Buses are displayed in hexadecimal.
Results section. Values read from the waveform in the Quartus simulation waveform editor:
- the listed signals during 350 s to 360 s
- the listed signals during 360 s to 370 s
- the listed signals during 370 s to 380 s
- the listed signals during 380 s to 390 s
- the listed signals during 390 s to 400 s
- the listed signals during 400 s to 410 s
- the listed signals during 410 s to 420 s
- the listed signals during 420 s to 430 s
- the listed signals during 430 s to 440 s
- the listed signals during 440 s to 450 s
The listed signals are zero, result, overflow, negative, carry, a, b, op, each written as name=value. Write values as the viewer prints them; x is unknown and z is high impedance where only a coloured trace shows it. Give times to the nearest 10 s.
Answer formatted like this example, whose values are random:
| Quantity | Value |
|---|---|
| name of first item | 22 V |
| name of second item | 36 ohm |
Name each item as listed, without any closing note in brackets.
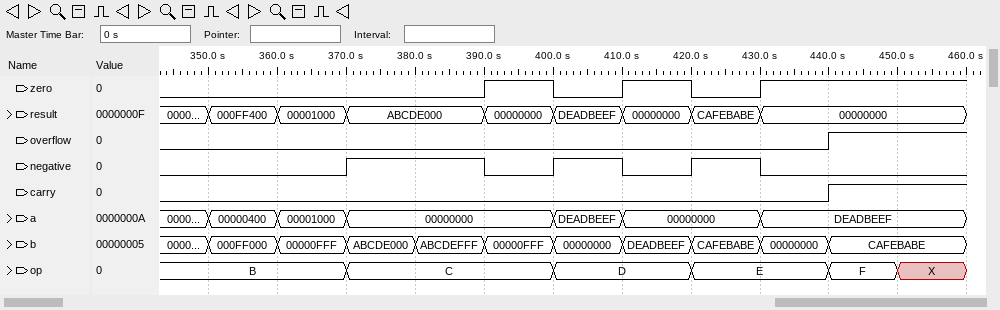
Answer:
| Quantity | Value |
|---|---|
| the listed signals during 350 s to 360 s | zero=0, result=000FF400, overflow=0, negative=0, carry=0, a=00000400, b=000FF000, op=B |
| the listed signals during 360 s to 370 s | zero=0, result=00001000, overflow=0, negative=0, carry=0, a=00001000, b=00000FFF, op=B |
| the listed signals during 370 s to 380 s | zero=0, result=ABCDE000, overflow=0, negative=1, carry=0, a=00000000, b=ABCDE000, op=C |
| the listed signals during 380 s to 390 s | zero=0, result=ABCDE000, overflow=0, negative=1, carry=0, a=00000000, b=ABCDEFFF, op=C |
| the listed signals during 390 s to 400 s | zero=1, result=00000000, overflow=0, negative=0, carry=0, a=00000000, b=00000FFF, op=C |
| the listed signals during 400 s to 410 s | zero=0, result=DEADBEEF, overflow=0, negative=1, carry=0, a=DEADBEEF, b=00000000, op=D |
| the listed signals during 410 s to 420 s | zero=1, result=00000000, overflow=0, negative=0, carry=0, a=00000000, b=DEADBEEF, op=D |
| the listed signals during 420 s to 430 s | zero=0, result=CAFEBABE, overflow=0, negative=1, carry=0, a=00000000, b=CAFEBABE, op=E |
| the listed signals during 430 s to 440 s | zero=1, result=00000000, overflow=0, negative=0, carry=0, a=DEADBEEF, b=00000000, op=E |
| the listed signals during 440 s to 450 s | zero=1, result=00000000, overflow=1, negative=0, carry=1, a=DEADBEEF, b=CAFEBABE, op=F |
